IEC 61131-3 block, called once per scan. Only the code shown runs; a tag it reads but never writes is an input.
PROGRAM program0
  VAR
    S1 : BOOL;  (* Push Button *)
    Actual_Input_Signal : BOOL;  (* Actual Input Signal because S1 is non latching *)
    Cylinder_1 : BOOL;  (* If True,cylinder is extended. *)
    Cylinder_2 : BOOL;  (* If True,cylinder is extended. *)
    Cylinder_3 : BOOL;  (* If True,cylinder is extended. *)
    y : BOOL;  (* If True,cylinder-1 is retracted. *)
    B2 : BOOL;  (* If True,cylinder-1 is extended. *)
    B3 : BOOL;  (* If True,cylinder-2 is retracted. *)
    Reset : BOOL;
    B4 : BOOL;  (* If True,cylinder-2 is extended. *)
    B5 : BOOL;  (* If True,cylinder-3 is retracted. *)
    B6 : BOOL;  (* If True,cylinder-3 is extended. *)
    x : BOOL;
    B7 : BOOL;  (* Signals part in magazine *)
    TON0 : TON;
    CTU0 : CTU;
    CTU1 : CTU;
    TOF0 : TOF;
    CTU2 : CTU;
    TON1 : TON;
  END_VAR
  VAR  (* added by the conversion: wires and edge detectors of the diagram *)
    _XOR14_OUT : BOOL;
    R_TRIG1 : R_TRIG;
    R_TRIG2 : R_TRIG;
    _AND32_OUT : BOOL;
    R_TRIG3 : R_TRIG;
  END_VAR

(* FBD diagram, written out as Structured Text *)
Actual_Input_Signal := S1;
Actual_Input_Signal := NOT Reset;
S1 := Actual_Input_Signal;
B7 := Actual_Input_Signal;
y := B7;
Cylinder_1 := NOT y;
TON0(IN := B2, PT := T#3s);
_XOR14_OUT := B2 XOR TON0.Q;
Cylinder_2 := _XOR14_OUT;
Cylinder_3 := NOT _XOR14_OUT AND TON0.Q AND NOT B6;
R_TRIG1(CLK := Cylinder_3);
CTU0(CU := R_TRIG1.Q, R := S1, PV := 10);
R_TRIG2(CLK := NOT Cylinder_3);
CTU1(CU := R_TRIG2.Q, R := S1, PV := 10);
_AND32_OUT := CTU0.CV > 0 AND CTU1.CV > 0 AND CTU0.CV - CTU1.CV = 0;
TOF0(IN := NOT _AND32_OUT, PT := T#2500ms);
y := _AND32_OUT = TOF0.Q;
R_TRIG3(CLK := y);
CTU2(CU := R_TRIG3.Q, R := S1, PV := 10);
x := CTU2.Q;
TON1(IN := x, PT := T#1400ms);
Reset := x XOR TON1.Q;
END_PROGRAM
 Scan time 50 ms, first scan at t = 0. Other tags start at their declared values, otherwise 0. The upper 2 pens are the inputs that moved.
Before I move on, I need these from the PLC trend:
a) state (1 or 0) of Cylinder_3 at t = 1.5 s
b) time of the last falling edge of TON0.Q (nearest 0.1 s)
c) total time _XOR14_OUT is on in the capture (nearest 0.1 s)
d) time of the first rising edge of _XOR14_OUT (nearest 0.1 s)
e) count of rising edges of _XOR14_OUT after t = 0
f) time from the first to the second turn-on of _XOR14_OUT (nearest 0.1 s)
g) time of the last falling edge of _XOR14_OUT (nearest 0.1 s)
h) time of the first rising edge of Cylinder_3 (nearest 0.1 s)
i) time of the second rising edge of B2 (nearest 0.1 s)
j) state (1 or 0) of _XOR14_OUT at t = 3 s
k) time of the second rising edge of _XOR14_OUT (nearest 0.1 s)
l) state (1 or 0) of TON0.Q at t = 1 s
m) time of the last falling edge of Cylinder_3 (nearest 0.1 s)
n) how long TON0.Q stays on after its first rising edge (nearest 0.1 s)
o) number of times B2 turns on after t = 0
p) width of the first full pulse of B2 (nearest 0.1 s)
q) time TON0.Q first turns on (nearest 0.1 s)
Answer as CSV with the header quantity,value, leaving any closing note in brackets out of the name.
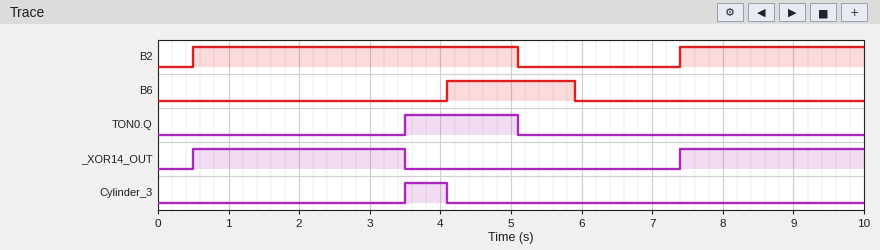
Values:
quantity,value
state (1 or 0) of Cylinder_3 at t = 1.5 s,0
time of the last falling edge of TON0.Q,5.1 s
total time _XOR14_OUT is on in the capture,5.6 s
time of the first rising edge of _XOR14_OUT,0.5 s
count of rising edges of _XOR14_OUT after t = 0,2
time from the first to the second turn-on of _XOR14_OUT,6.9 s
time of the last falling edge of _XOR14_OUT,3.5 s
time of the first rising edge of Cylinder_3,3.5 s
time of the second rising edge of B2,7.4 s
state (1 or 0) of _XOR14_OUT at t = 3 s,1
time of the second rising edge of _XOR14_OUT,7.4 s
state (1 or 0) of TON0.Q at t = 1 s,0
time of the last falling edge of Cylinder_3,4.1 s
how long TON0.Q stays on after its first rising edge,1.6 s
number of times B2 turns on after t = 0,2
width of the first full pulse of B2,4.6 s
time TON0.Q first turns on,3.5 s
